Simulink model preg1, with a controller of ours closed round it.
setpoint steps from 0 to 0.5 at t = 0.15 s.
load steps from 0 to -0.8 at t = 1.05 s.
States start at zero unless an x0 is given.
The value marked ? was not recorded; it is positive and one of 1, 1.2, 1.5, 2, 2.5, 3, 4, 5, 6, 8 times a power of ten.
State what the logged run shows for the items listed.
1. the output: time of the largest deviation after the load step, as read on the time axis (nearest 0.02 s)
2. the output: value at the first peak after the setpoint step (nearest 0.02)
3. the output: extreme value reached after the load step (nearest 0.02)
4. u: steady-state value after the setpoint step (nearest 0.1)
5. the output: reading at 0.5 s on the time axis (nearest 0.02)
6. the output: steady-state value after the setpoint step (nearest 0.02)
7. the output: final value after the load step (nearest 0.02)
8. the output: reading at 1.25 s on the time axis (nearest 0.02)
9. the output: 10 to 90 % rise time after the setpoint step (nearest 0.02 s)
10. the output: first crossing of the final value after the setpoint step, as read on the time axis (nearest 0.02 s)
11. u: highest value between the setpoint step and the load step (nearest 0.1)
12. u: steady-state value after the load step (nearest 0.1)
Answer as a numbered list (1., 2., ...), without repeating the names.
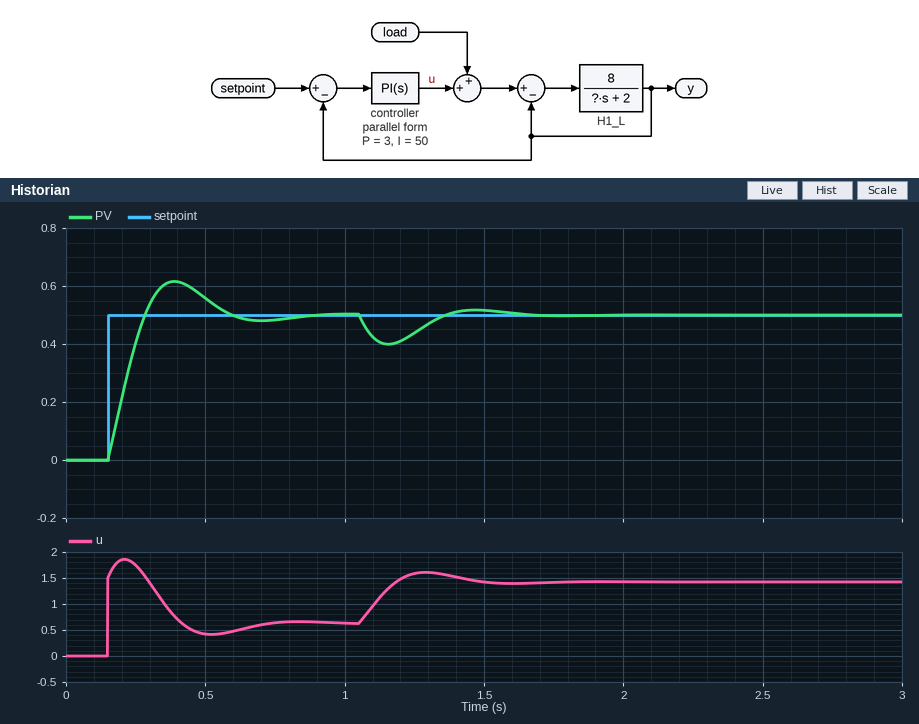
1. 1.16 s
2. 0.62
3. 0.40
4. 0.6
5. 0.56
6. 0.50
7. 0.50
8. 0.44
9. 0.10 s
10. 0.28 s
11. 1.9
12. 1.4
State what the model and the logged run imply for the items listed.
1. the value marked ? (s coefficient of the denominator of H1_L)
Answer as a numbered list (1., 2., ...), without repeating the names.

1. 3
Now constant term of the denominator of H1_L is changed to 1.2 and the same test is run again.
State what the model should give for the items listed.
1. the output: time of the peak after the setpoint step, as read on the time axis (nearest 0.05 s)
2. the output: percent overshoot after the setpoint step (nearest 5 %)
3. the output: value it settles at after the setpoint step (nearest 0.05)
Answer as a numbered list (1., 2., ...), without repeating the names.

1. 0.40 s
2. 25 %
3. 0.50
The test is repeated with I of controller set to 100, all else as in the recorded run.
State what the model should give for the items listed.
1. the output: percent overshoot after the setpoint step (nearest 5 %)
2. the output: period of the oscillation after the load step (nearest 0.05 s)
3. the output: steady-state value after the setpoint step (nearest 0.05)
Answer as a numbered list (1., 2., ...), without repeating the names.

1. 35 %
2. 0.40 s
3. 0.50
